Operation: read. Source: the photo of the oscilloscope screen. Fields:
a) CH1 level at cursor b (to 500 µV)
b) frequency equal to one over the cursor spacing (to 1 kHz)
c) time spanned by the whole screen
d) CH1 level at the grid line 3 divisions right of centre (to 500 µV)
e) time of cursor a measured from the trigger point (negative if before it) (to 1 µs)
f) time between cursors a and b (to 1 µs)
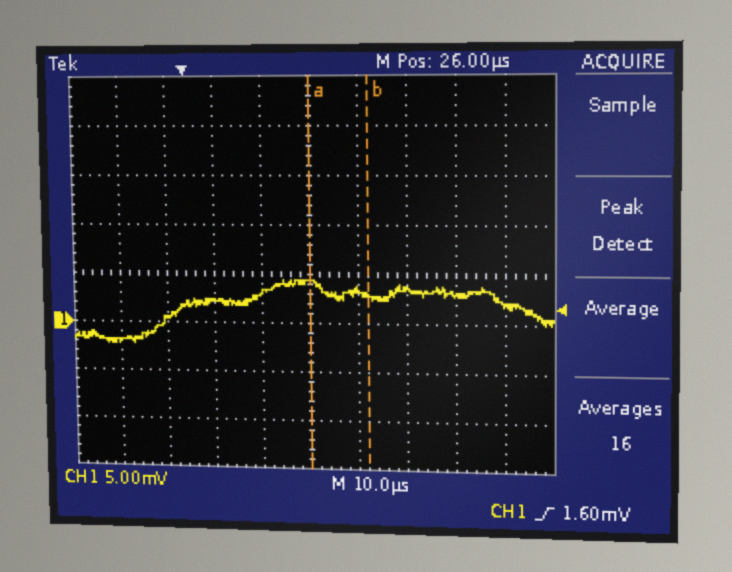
3.0 mV
83 kHz
100 µs
3.0 mV
+26 µs
12 µs
